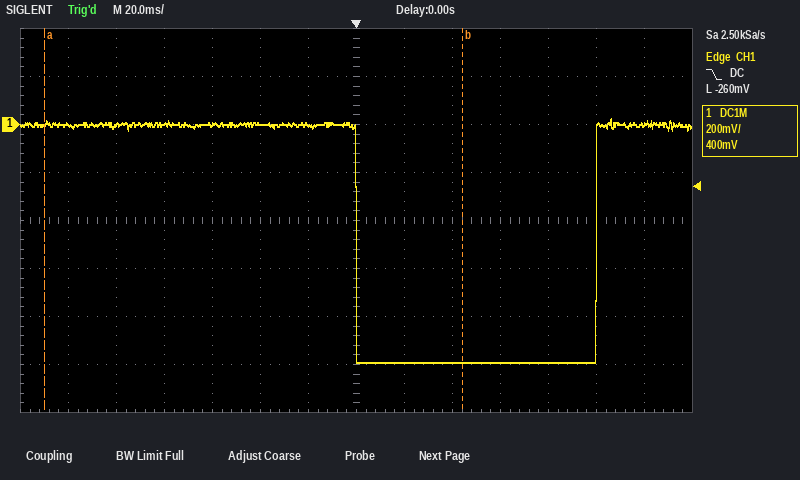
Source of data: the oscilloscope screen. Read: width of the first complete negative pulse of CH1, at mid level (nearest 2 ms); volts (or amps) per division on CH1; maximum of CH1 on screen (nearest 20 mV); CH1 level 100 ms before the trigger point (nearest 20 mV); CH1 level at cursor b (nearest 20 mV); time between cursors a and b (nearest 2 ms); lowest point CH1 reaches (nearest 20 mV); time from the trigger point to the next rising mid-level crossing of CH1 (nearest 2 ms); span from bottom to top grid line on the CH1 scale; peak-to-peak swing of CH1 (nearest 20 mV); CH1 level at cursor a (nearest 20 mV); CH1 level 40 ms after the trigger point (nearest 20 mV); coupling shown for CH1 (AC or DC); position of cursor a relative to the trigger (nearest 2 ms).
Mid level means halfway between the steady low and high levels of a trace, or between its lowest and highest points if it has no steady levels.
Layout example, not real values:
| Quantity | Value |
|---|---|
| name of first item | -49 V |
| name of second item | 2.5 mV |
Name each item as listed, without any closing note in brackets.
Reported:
| Quantity | Value |
|---|---|
| width of the first complete negative pulse of CH1, at mid level | 100 ms |
| volts (or amps) per division on CH1 | 200 mV |
| maximum of CH1 on screen | 20 mV |
| CH1 level 100 ms before the trigger point | 0 mV |
| CH1 level at cursor b | -1.00 V |
| time between cursors a and b | 174 ms |
| lowest point CH1 reaches | -1.00 V |
| time from the trigger point to the next rising mid-level crossing of CH1 | 100 ms |
| span from bottom to top grid line on the CH1 scale | 1.6 V |
| peak-to-peak swing of CH1 | 1.02 V |
| CH1 level at cursor a | 0 mV |
| CH1 level 40 ms after the trigger point | -1.00 V |
| coupling shown for CH1 | DC |
| position of cursor a relative to the trigger | -130 ms |
